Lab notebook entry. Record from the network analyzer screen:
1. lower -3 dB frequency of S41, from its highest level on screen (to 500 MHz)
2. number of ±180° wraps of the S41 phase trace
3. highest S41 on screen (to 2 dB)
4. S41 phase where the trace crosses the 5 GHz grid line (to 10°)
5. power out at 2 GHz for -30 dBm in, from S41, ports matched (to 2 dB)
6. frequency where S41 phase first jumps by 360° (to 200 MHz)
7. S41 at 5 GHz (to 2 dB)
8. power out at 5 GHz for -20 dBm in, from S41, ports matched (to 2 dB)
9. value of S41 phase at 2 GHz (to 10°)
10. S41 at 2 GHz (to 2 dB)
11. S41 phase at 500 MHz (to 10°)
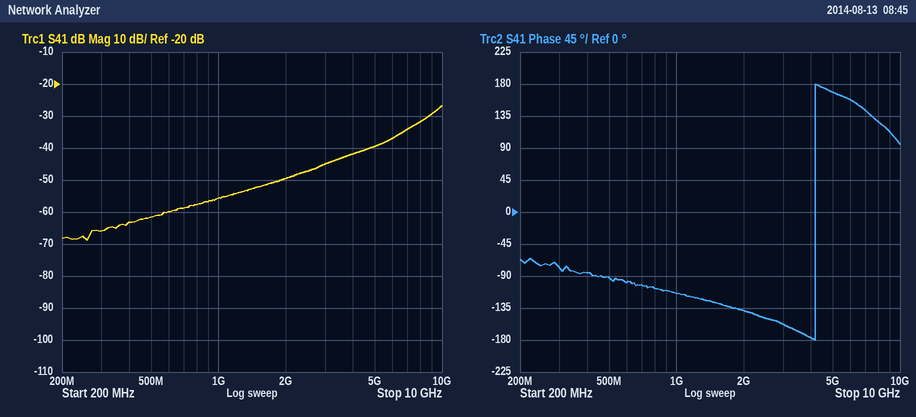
9.0 GHz
1
-26 dB
170°
-80 dBm
4.2 GHz
-40 dB
-60 dBm
-140°
-50 dB
-90°
